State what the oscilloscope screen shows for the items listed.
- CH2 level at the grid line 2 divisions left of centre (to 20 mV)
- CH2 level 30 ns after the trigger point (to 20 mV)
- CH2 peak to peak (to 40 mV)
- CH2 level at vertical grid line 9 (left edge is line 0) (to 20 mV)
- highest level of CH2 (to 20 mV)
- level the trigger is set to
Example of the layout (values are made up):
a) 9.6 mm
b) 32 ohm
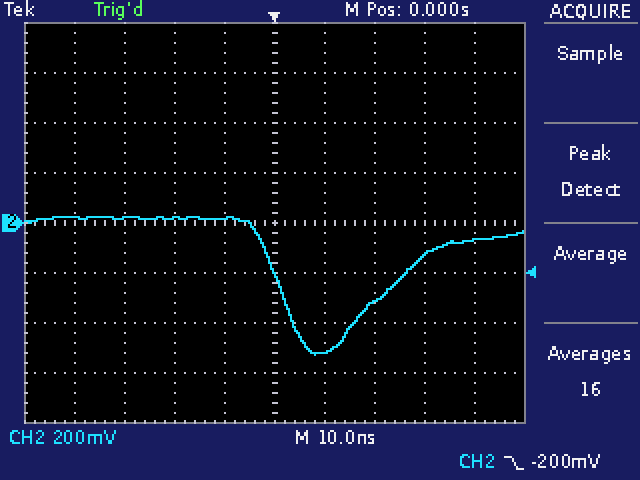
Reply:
a) 20 mV
b) -120 mV
c) 560 mV
d) -60 mV
e) 20 mV
f) -200 mV
